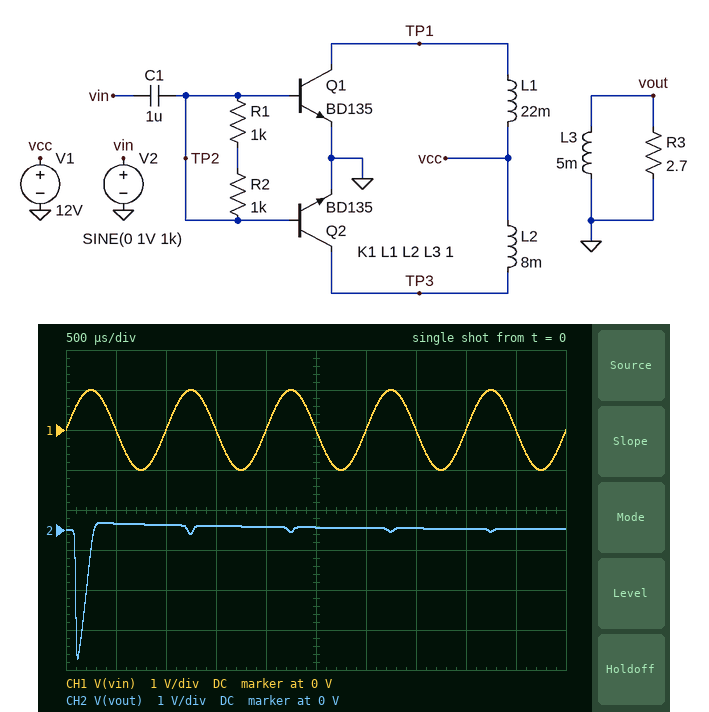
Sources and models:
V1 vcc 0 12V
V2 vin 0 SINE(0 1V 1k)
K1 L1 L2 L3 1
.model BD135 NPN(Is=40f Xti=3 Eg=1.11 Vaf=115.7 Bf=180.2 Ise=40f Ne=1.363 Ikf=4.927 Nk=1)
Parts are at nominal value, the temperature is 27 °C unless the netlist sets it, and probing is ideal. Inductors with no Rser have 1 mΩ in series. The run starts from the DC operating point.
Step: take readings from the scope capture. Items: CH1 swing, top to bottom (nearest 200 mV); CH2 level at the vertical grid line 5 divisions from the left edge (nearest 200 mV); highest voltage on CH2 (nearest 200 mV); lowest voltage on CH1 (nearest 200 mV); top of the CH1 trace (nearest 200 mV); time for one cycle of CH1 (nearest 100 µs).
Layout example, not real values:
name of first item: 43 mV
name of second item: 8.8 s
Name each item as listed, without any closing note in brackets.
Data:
CH1 swing, top to bottom: 2.0 V
CH2 level at the vertical grid line 5 divisions from the left edge: 0 V
highest voltage on CH2: 200 mV
lowest voltage on CH1: -1.0 V
top of the CH1 trace: 1.0 V
time for one cycle of CH1: 1.0 ms
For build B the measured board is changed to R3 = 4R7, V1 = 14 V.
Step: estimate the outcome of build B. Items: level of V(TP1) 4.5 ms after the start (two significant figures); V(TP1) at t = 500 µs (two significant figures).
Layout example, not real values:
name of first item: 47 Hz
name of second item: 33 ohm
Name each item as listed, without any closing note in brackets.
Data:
level of V(TP1) 4.5 ms after the start: 14 V
V(TP1) at t = 500 µs: 15 V
